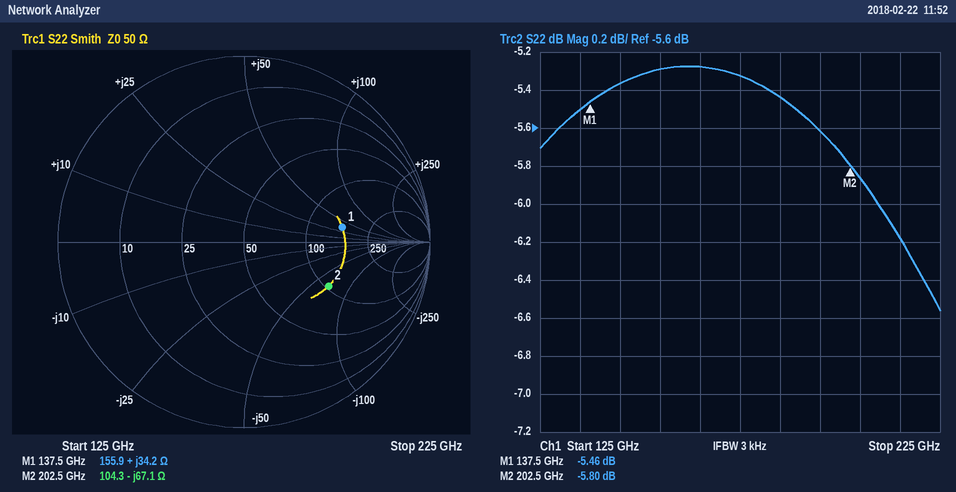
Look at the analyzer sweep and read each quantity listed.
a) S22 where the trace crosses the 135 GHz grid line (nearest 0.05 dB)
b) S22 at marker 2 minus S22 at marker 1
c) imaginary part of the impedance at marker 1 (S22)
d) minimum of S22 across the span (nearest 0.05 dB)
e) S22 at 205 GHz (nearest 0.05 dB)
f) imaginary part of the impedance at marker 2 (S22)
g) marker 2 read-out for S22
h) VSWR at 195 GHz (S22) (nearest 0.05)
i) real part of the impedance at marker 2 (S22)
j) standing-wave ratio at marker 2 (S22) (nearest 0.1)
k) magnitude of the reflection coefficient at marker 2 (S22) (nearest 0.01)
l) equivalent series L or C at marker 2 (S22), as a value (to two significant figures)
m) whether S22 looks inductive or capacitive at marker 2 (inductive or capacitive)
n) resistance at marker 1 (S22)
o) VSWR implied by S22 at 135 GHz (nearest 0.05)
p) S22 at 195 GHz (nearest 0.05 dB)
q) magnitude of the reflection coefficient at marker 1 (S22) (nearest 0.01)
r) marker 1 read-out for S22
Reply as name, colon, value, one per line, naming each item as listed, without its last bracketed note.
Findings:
S22 where the trace crosses the 135 GHz grid line: -5.50 dB
S22 at marker 2 minus S22 at marker 1: -0.34 dB
imaginary part of the impedance at marker 1: +34.2 Ω
minimum of S22 across the span: -6.55 dB
S22 at 205 GHz: -5.85 dB
imaginary part of the impedance at marker 2: -67.1 Ω
marker 2 read-out for S22: -5.80 dB
VSWR at 195 GHz (S22): 3.20
real part of the impedance at marker 2: 104.3 Ω
standing-wave ratio at marker 2 (S22): 3.1
magnitude of the reflection coefficient at marker 2 (S22): 0.51
equivalent series L or C at marker 2 (S22), as a value: 12 fF
whether S22 looks inductive or capacitive at marker 2: capacitive
resistance at marker 1: 155.9 Ω
VSWR implied by S22 at 135 GHz: 3.25
S22 at 195 GHz: -5.60 dB
magnitude of the reflection coefficient at marker 1 (S22): 0.53
marker 1 read-out for S22: -5.46 dB
